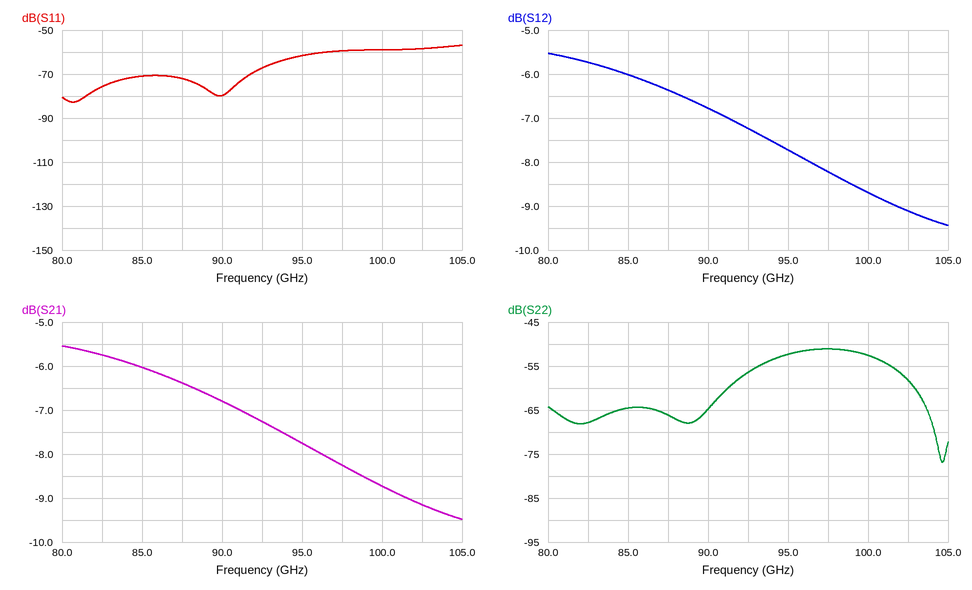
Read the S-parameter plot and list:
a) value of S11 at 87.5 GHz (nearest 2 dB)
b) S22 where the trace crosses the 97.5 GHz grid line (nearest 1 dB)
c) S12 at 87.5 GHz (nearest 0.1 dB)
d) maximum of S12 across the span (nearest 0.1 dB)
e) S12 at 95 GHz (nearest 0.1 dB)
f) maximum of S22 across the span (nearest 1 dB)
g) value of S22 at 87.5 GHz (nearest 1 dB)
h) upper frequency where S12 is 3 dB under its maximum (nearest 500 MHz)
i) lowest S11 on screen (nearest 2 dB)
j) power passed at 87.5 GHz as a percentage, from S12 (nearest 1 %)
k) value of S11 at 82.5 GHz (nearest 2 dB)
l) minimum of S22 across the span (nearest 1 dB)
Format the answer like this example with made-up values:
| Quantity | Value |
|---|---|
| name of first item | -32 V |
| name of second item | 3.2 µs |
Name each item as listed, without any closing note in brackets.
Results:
| Quantity | Value |
|---|---|
| value of S11 at 87.5 GHz | -72 dB |
| S22 where the trace crosses the 97.5 GHz grid line | -51 dB |
| S12 at 87.5 GHz | -6.4 dB |
| maximum of S12 across the span | -5.5 dB |
| S12 at 95 GHz | -7.7 dB |
| maximum of S22 across the span | -51 dB |
| value of S22 at 87.5 GHz | -66 dB |
| upper frequency where S12 is 3 dB under its maximum | 99.0 GHz |
| lowest S11 on screen | -82 dB |
| power passed at 87.5 GHz as a percentage, from S12 | 23 % |
| value of S11 at 82.5 GHz | -76 dB |
| minimum of S22 across the span | -77 dB |
